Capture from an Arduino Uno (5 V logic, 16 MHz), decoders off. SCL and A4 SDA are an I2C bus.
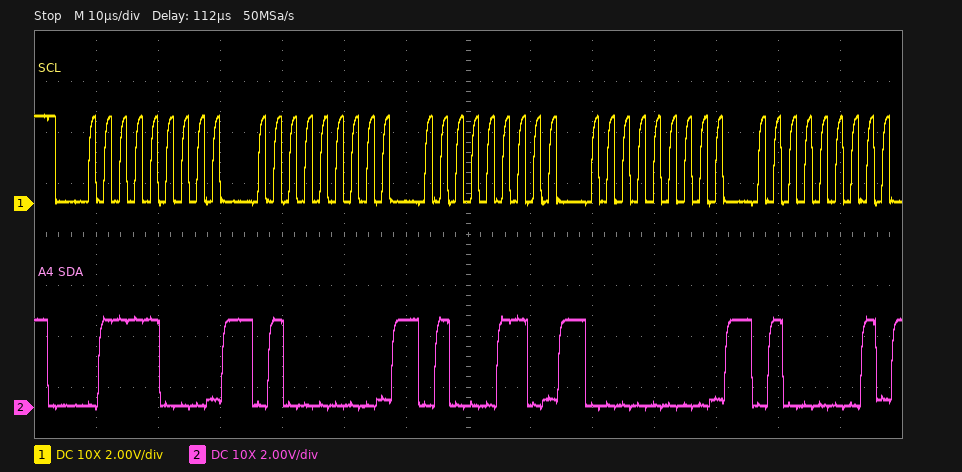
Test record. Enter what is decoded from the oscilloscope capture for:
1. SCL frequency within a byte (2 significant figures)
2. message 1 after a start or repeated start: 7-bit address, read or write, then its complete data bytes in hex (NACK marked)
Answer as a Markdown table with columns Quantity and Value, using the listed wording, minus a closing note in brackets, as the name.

| Quantity | Value |
|---|---|
| SCL frequency within a byte | 400 kHz |
| message 1 after a start or repeated start: 7-bit address, read or write, then its complete data bytes in hex | 0x3C write: 40 46 00 41 |
